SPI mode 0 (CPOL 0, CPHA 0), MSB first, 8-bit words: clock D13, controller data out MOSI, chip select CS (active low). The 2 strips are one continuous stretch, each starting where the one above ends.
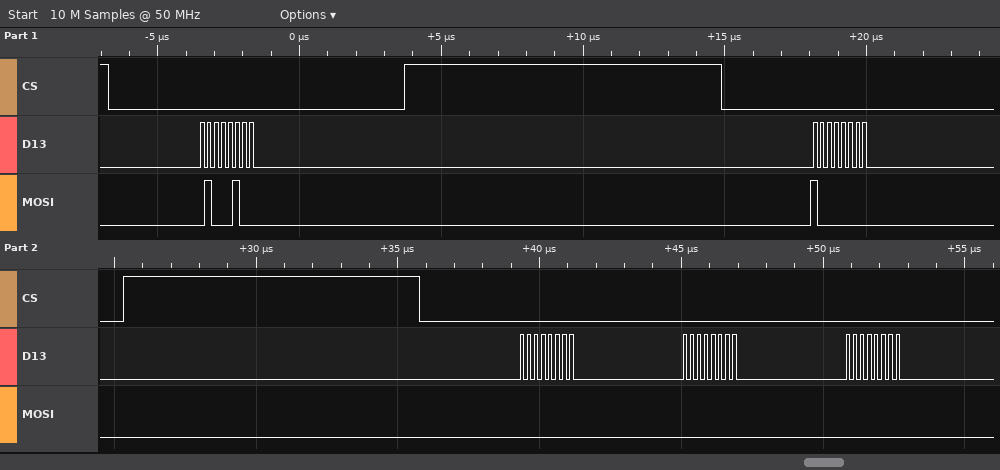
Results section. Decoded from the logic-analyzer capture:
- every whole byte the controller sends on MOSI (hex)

44 80 00 00 00
